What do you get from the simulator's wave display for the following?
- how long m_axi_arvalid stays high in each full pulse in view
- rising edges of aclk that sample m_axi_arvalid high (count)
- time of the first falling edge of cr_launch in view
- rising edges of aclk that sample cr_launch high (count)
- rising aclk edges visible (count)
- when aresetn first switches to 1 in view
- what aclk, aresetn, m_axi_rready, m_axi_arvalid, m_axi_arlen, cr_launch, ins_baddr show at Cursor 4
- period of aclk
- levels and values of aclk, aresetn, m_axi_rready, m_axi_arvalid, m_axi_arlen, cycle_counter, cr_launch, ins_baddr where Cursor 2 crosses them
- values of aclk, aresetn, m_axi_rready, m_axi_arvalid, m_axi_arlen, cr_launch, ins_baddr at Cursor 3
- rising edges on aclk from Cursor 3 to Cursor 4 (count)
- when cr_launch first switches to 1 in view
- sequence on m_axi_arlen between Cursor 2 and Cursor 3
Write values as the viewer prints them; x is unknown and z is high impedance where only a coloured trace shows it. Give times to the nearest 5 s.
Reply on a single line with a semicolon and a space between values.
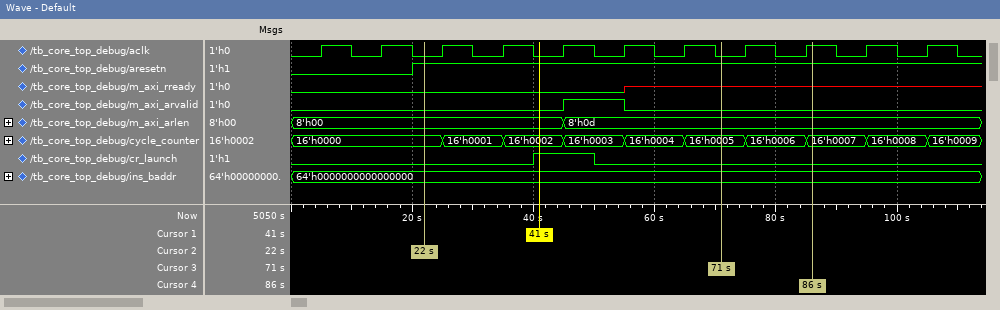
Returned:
10 s; 1; 50 s; 1; 11; 20 s; aclk=1, aresetn=1, m_axi_rready=x, m_axi_arvalid=0, m_axi_arlen=8'h0d, cr_launch=0, ins_baddr=64'h0000000000000000; 10 s; aclk=0, aresetn=1, m_axi_rready=0, m_axi_arvalid=0, m_axi_arlen=8'h00, cycle_counter=16'h0000, cr_launch=0, ins_baddr=64'h0000000000000000; aclk=0, aresetn=1, m_axi_rready=x, m_axi_arvalid=0, m_axi_arlen=8'h0d, cr_launch=0, ins_baddr=64'h0000000000000000; 2; 40 s; 8'h00, 8'h0d
